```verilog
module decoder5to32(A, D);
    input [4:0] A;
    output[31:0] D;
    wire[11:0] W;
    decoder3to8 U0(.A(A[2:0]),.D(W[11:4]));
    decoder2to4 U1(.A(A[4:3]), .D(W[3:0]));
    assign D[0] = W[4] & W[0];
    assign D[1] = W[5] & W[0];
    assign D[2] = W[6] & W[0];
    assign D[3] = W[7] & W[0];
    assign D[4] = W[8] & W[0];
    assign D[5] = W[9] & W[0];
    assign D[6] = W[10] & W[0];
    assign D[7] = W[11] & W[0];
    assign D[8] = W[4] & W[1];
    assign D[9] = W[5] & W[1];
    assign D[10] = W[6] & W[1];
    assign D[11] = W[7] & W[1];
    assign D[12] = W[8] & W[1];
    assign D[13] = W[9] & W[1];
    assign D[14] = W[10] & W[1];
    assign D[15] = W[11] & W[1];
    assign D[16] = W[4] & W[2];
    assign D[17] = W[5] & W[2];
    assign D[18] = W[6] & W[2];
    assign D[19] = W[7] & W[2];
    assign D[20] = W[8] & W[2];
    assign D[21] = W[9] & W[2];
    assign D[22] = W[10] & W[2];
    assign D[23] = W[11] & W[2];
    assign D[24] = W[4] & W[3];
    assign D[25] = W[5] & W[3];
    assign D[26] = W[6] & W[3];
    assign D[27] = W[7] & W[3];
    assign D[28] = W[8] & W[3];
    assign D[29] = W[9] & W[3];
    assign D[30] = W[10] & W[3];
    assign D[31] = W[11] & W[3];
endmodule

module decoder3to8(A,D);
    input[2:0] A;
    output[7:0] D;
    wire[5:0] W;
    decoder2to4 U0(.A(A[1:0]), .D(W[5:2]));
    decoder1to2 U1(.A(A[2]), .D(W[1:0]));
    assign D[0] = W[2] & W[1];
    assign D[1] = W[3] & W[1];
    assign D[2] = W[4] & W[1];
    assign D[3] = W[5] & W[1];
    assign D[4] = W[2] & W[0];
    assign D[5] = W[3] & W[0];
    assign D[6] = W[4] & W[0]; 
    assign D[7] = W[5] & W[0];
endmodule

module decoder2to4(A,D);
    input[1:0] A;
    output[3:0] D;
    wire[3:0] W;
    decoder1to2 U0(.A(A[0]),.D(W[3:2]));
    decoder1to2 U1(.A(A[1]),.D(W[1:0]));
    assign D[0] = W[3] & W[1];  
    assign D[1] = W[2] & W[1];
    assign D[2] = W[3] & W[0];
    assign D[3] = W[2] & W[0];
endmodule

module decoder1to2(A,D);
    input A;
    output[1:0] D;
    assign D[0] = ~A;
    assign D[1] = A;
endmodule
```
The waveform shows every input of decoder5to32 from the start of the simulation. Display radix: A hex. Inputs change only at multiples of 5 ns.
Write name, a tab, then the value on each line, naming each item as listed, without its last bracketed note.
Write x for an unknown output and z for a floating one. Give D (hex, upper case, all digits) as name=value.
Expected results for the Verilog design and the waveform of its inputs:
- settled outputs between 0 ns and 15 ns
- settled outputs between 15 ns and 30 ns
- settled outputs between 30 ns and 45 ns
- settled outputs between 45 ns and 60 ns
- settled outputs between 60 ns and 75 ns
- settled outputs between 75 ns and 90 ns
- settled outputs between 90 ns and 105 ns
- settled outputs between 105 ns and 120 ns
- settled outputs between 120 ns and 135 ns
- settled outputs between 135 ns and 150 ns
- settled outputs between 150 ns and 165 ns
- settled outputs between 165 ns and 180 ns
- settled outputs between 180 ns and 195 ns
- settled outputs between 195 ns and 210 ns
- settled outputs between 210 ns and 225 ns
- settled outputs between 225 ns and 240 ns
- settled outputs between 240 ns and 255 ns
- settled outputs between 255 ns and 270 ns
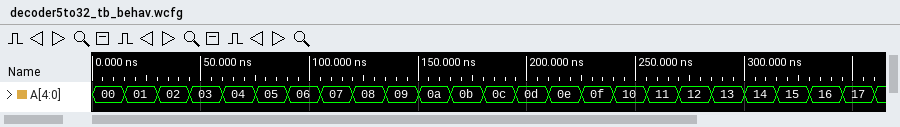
settled outputs between 0 ns and 15 ns	D=80000000
settled outputs between 15 ns and 30 ns	D=40000000
settled outputs between 30 ns and 45 ns	D=20000000
settled outputs between 45 ns and 60 ns	D=10000000
settled outputs between 60 ns and 75 ns	D=08000000
settled outputs between 75 ns and 90 ns	D=04000000
settled outputs between 90 ns and 105 ns	D=02000000
settled outputs between 105 ns and 120 ns	D=01000000
settled outputs between 120 ns and 135 ns	D=00800000
settled outputs between 135 ns and 150 ns	D=00400000
settled outputs between 150 ns and 165 ns	D=00200000
settled outputs between 165 ns and 180 ns	D=00100000
settled outputs between 180 ns and 195 ns	D=00080000
settled outputs between 195 ns and 210 ns	D=00040000
settled outputs between 210 ns and 225 ns	D=00020000
settled outputs between 225 ns and 240 ns	D=00010000
settled outputs between 240 ns and 255 ns	D=00008000
settled outputs between 255 ns and 270 ns	D=00004000
